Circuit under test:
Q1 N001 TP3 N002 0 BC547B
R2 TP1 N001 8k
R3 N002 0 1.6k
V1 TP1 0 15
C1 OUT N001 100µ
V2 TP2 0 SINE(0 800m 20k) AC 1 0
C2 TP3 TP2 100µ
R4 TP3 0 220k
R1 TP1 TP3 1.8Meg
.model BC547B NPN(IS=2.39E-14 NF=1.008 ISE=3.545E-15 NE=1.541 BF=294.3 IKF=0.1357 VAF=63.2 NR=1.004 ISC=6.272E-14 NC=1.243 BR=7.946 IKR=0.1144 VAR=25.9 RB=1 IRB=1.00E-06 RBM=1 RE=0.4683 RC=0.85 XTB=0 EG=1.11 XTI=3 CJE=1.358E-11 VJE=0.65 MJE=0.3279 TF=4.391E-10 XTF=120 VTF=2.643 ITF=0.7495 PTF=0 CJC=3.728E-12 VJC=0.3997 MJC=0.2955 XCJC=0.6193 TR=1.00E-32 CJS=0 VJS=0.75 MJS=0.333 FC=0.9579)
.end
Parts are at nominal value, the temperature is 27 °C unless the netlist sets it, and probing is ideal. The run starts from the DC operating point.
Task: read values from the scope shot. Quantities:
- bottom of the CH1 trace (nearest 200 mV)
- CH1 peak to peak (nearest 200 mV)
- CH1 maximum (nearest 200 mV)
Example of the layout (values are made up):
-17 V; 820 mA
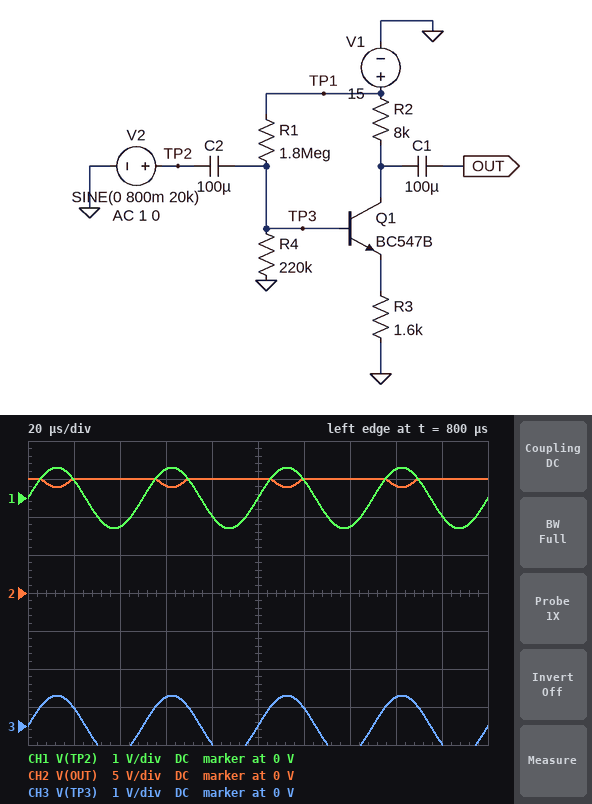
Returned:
-800 mV; 1.6 V; 800 mV
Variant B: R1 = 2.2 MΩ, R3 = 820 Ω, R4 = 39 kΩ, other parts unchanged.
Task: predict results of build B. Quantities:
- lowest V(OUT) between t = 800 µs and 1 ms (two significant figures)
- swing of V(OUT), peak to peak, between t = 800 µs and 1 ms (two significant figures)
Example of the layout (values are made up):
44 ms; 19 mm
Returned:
13 V; 2.0 V
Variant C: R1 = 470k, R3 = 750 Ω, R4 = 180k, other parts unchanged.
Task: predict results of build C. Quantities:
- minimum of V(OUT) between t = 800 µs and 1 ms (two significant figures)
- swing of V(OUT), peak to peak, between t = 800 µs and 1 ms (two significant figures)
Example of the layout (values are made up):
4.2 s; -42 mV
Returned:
13 V; 2.1 V
